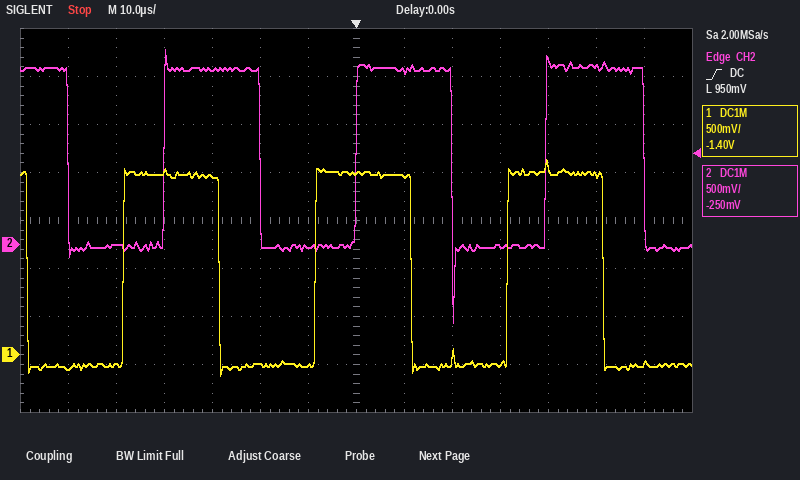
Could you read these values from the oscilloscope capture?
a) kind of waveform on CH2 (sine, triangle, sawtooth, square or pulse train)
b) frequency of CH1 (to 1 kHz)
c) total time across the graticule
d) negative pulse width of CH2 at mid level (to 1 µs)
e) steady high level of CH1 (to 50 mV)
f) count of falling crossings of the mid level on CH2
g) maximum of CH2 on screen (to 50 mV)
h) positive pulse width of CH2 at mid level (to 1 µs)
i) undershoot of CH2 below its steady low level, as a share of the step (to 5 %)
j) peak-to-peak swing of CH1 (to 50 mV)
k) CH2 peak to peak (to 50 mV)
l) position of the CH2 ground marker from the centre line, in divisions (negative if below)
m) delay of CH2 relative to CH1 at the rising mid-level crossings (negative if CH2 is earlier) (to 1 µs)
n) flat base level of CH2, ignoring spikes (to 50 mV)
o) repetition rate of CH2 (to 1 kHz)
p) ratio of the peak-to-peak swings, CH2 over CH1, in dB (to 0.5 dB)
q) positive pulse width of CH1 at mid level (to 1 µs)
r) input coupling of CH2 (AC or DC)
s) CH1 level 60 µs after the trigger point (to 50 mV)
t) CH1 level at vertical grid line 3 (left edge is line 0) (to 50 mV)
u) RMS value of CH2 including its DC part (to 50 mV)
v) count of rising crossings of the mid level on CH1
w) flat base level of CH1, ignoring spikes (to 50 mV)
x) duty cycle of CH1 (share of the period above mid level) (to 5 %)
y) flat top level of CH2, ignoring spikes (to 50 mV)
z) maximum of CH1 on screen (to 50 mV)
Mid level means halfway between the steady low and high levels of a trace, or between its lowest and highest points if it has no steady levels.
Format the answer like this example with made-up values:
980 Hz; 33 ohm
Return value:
square; 25 kHz; 140 µs; 20 µs; 1.90 V; 4; 2.05 V; 20 µs; 40 %; 2.25 V; 2.85 V; -0.5 div; +8 µs; -50 mV; 25 kHz; 2.0 dB; 20 µs; DC; -100 mV; 1.90 V; 1.30 V; 3; -100 mV; 50 %; 1.85 V; 2.05 V
